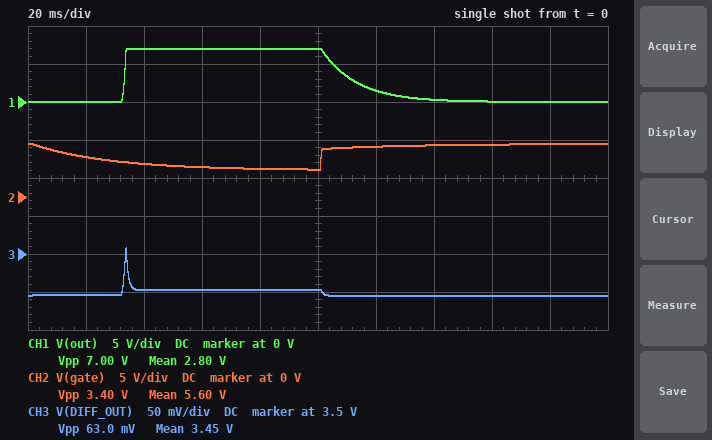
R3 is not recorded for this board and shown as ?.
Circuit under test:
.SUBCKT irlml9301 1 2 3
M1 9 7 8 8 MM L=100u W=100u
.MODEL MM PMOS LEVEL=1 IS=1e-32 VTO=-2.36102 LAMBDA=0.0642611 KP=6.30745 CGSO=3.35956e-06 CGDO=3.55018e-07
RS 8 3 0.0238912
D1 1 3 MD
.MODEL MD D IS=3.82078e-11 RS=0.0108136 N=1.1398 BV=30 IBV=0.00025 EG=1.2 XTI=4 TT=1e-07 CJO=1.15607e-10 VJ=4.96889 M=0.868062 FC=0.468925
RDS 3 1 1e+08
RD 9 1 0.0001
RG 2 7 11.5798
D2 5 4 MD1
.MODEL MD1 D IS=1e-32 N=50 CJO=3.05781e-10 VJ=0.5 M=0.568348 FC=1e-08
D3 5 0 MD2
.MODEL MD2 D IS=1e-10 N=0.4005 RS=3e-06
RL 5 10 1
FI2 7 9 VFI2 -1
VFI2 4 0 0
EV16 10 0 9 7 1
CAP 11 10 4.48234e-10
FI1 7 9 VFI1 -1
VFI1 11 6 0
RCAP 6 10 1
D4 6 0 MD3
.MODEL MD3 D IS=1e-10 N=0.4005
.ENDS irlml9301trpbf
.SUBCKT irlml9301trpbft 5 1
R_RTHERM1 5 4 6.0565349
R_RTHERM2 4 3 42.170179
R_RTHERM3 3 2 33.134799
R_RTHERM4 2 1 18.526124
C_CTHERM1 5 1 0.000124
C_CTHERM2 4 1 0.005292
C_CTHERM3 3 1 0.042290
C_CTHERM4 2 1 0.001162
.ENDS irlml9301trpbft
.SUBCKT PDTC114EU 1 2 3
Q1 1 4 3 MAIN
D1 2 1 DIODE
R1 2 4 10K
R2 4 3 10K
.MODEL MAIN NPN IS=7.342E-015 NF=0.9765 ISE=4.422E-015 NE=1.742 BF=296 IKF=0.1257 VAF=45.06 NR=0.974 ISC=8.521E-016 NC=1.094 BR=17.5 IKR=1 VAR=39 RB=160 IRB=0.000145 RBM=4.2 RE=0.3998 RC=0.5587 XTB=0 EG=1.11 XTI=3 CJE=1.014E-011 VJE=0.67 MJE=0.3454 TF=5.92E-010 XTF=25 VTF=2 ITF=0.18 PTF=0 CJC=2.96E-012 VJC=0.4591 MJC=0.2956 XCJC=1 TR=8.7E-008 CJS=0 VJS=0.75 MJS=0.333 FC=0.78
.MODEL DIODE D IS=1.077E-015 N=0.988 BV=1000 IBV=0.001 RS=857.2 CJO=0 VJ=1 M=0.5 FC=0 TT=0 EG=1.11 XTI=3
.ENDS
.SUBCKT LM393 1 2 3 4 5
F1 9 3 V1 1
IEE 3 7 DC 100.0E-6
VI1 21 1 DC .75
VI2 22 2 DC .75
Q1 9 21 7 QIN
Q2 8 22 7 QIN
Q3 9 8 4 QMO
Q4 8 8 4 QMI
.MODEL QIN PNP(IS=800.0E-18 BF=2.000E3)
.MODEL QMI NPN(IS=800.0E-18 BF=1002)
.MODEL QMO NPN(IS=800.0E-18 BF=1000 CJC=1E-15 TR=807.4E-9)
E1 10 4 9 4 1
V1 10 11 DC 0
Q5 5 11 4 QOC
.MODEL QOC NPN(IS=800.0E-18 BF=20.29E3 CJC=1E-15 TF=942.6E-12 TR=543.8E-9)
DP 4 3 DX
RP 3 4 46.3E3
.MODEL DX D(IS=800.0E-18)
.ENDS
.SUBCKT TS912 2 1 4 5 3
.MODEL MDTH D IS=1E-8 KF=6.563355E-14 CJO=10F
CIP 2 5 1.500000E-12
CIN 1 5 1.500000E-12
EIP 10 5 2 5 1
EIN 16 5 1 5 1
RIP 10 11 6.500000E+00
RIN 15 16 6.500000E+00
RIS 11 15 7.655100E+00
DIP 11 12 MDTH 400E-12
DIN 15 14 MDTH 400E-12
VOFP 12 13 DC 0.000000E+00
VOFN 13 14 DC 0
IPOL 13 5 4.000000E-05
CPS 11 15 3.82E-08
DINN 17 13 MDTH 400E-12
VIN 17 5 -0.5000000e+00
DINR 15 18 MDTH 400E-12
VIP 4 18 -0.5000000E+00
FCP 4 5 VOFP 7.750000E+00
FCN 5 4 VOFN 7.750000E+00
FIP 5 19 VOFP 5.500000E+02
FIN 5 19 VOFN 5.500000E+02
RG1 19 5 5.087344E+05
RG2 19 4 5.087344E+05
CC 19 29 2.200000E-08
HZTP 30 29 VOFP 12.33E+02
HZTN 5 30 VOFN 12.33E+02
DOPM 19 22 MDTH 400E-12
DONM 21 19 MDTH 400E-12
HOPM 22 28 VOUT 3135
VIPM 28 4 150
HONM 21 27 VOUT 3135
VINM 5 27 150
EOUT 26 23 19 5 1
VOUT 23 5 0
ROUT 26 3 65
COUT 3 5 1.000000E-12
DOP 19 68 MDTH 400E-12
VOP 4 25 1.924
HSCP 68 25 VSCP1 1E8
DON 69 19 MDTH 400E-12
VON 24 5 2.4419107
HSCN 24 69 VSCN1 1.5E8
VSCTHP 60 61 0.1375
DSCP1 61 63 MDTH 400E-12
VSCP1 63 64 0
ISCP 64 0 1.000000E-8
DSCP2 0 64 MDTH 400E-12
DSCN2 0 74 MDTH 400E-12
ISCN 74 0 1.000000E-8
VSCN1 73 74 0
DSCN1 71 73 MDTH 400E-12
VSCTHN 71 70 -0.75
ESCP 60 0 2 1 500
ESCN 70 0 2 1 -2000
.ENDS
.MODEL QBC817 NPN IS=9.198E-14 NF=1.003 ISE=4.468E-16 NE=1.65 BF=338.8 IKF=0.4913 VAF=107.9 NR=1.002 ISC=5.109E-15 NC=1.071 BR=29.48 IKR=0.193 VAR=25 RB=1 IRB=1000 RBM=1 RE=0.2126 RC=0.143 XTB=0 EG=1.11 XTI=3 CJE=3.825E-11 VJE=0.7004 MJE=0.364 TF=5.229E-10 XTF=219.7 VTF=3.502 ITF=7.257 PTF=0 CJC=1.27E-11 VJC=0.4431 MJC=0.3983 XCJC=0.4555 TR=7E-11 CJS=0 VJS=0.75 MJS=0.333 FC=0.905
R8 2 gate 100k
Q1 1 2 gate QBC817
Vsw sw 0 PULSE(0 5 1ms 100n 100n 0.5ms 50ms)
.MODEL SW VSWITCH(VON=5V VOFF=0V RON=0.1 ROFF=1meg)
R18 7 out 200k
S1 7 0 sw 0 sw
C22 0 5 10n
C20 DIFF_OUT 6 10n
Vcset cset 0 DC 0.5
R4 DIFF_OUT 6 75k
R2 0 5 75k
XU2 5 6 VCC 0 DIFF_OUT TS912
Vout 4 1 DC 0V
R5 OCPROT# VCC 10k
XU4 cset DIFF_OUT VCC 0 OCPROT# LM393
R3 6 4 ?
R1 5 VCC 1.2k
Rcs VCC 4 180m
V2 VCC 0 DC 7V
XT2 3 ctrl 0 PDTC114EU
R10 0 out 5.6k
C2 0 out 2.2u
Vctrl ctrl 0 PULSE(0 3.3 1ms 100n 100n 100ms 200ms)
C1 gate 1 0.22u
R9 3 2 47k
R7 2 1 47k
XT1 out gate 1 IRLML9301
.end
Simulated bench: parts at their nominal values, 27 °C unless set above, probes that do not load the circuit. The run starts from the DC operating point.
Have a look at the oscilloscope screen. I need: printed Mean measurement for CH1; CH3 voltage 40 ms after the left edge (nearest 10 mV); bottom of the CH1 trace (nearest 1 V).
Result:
2.80 V
3.45 V
0 V
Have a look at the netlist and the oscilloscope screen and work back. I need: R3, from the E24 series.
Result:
2.4 kΩ
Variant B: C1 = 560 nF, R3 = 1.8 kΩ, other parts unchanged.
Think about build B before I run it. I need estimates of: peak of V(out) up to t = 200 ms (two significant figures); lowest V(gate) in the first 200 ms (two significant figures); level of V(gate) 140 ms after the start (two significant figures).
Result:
7.0 V
4.3 V
6.6 V
